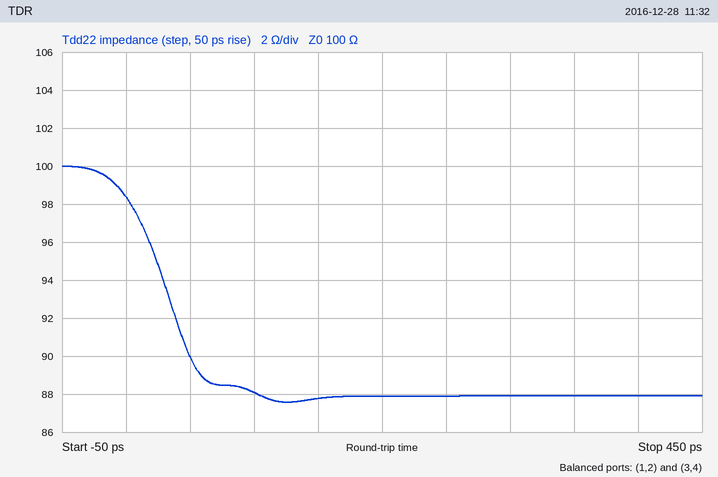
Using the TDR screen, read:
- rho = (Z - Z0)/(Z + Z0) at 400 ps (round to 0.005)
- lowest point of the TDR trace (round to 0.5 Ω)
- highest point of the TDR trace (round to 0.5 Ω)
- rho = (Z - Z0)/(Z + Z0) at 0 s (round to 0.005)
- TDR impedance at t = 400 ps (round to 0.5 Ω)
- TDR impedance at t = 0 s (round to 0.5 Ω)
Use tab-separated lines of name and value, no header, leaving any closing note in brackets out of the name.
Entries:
rho = (Z - Z0)/(Z + Z0) at 400 ps	-0.065
lowest point of the TDR trace	87.5 Ω
highest point of the TDR trace	100.0 Ω
rho = (Z - Z0)/(Z + Z0) at 0 s	-0.010
TDR impedance at t = 400 ps	88.0 Ω
TDR impedance at t = 0 s	98.5 Ω
